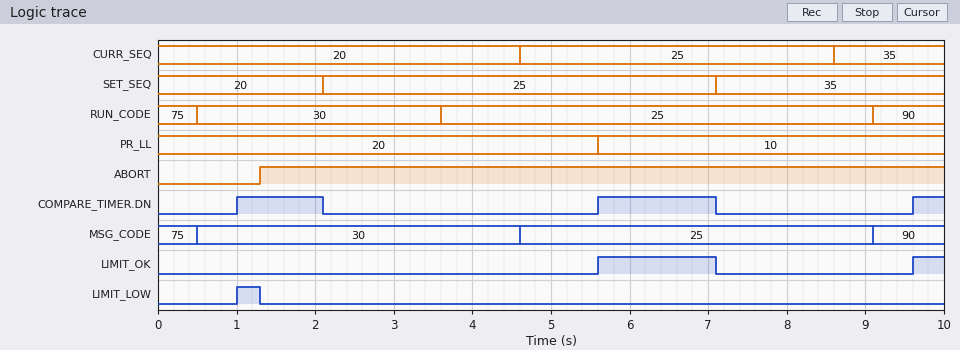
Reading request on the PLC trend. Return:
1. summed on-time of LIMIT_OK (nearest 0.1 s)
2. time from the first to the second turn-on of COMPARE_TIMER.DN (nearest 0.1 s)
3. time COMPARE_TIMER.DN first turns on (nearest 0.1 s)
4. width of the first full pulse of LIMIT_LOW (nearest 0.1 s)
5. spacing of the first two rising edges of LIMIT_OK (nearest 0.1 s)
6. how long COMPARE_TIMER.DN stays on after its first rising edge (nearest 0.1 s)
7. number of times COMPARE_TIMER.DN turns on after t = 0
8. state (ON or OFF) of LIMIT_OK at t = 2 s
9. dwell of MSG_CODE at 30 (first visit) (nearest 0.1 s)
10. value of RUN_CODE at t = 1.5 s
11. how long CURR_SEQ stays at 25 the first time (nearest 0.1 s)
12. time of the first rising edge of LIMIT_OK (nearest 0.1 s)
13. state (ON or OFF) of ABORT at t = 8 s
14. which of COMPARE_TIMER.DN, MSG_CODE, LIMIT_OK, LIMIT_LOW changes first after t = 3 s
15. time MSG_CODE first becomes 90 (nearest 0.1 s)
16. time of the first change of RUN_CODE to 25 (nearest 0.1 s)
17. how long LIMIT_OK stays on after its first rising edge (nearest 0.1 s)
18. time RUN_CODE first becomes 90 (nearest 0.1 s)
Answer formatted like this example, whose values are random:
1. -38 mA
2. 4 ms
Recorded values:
1. 1.9 s
2. 4.6 s
3. 1.0 s
4. 0.3 s
5. 4.0 s
6. 1.1 s
7. 3
8. OFF
9. 4.1 s
10. 30
11. 4.0 s
12. 5.6 s
13. ON
14. MSG_CODE
15. 9.1 s
16. 3.6 s
17. 1.5 s
18. 9.1 s
